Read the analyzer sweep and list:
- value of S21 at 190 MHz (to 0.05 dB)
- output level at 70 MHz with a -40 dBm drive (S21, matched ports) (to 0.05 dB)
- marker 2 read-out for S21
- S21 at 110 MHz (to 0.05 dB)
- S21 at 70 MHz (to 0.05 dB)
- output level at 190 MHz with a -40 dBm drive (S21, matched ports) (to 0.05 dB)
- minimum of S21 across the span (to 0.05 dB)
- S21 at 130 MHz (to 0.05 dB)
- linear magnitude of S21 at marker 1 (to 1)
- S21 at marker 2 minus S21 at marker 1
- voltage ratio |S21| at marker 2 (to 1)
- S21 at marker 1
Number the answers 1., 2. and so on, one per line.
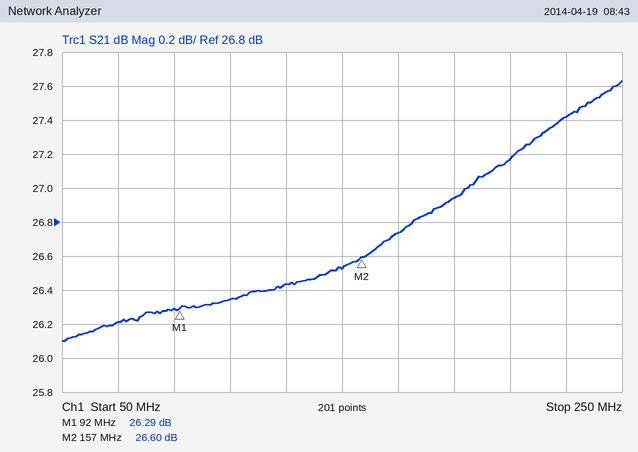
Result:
1. 26.95 dB
2. -13.80 dBm
3. 26.60 dB
4. 26.35 dB
5. 26.20 dB
6. -13.05 dBm
7. 26.10 dB
8. 26.45 dB
9. 21
10. 0.31 dB
11. 21
12. 26.29 dB
